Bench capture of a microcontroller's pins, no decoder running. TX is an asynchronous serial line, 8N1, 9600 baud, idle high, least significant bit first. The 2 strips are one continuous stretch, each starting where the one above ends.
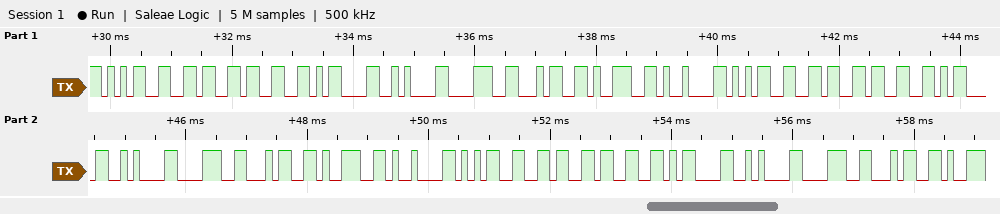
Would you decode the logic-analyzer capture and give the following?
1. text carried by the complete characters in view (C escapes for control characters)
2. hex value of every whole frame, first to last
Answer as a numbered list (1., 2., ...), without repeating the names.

1. "563\r\n849\t563\r\n849\t563\r\n84"
2. 0x35 0x36 0x33 0x0D 0x0A 0x38 0x34 0x39 0x09 0x35 0x36 0x33 0x0D 0x0A 0x38 0x34 0x39 0x09 0x35 0x36 0x33 0x0D 0x0A 0x38 0x34
